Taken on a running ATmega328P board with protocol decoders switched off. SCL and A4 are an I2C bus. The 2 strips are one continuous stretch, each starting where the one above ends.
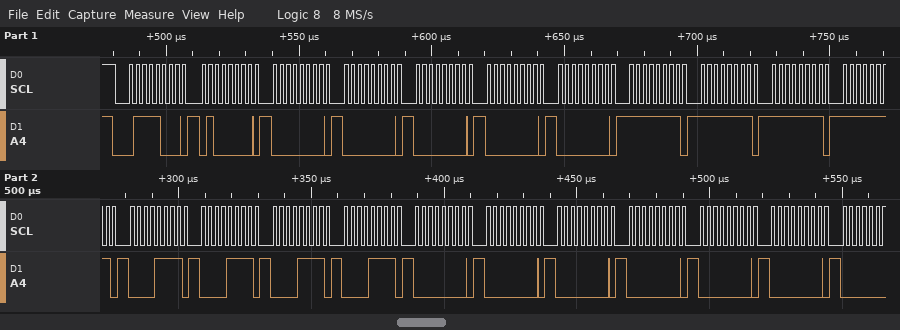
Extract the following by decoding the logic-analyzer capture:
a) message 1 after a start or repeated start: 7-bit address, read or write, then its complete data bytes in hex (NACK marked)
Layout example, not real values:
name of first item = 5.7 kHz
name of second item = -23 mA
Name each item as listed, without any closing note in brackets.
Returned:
message 1 after a start or repeated start: 7-bit address, read or write, then its complete data bytes in hex = 0x3C write: 40 00 00 00 00 00 FF FF FF FF 0F 0F 0F 0F 00 00 00 00 00 00
